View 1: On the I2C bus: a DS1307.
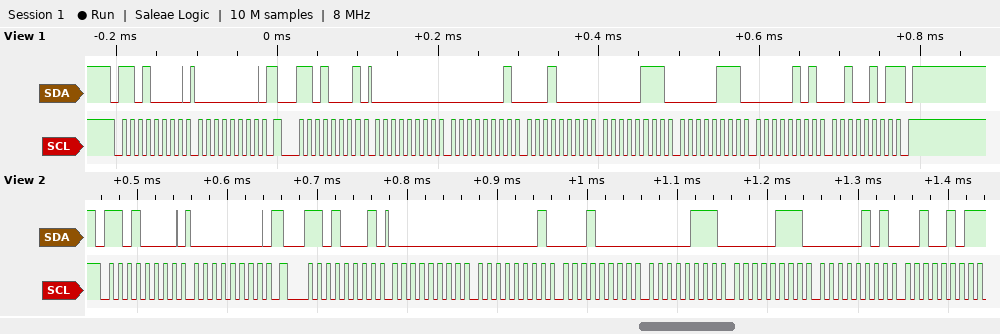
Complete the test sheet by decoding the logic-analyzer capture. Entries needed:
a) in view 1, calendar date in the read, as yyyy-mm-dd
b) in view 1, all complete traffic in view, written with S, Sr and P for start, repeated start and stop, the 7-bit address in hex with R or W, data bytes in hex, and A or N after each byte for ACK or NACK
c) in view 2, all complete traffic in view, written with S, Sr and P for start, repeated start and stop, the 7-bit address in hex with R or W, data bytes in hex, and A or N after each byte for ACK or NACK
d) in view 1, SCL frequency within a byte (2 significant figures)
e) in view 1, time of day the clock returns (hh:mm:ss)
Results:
2025-05-07
S 68W A 00 A Sr 68R A 00 A 01 A 10 A 07 A 07 A 05 A 25 N P
S 68W A 00 A Sr 68R A 00 A 01 A 10 A 07 A 07 A 05 A 25 N
100 kHz
10:01:00
